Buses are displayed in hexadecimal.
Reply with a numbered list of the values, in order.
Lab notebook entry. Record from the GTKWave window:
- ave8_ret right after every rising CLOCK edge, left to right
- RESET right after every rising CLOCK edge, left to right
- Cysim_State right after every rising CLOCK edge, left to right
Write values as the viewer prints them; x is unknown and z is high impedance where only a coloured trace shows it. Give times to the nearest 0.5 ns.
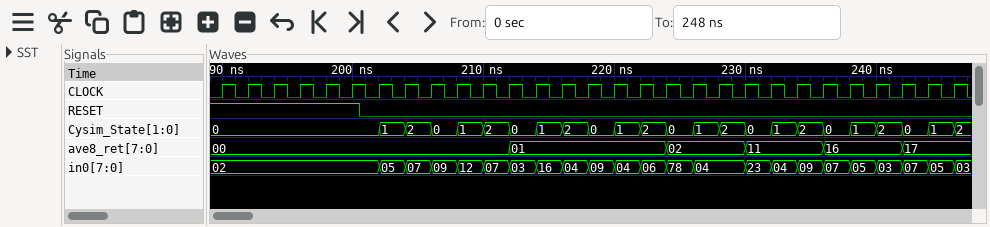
1. 00, 00, 00, 00, 00, 00, 00, 00, 00, 00, 00, 01, 01, 01, 01, 01, 01, 02, 02, 02, 11, 11, 11, 16, 16, 16, 17, 17, 17
2. 1 1 1 1 1 1 0 0 0 0 0 0 0 0 0 0 0 0 0 0 0 0 0 0 0 0 0 0 0
3. 0, 0, 0, 0, 0, 0, 1, 2, 0, 1, 2, 0, 1, 2, 0, 1, 2, 0, 1, 2, 0, 1, 2, 0, 1, 2, 0, 1, 2
